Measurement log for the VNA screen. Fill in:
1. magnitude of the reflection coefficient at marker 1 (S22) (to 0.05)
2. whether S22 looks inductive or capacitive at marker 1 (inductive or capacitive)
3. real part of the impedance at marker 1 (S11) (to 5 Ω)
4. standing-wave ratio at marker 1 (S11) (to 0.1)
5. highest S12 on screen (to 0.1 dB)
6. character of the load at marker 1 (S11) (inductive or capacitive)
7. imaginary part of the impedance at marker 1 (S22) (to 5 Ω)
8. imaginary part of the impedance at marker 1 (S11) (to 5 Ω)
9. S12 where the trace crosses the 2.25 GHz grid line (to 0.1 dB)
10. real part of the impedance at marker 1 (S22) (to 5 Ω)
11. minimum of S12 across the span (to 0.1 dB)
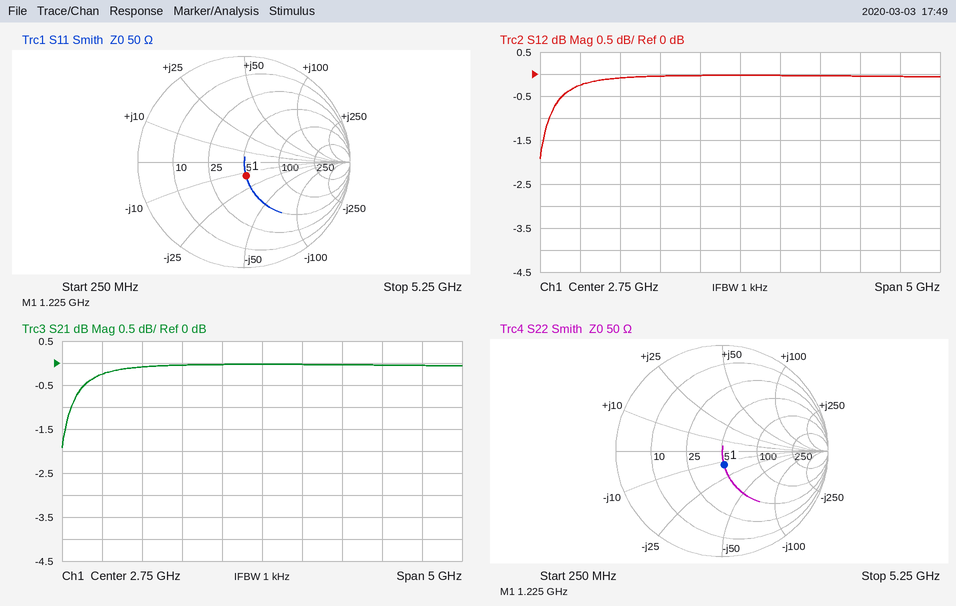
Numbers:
0.15
capacitive
50 Ω
1.3
0.0 dB
capacitive
-15 Ω
-15 Ω
0.0 dB
50 Ω
-1.9 dB
